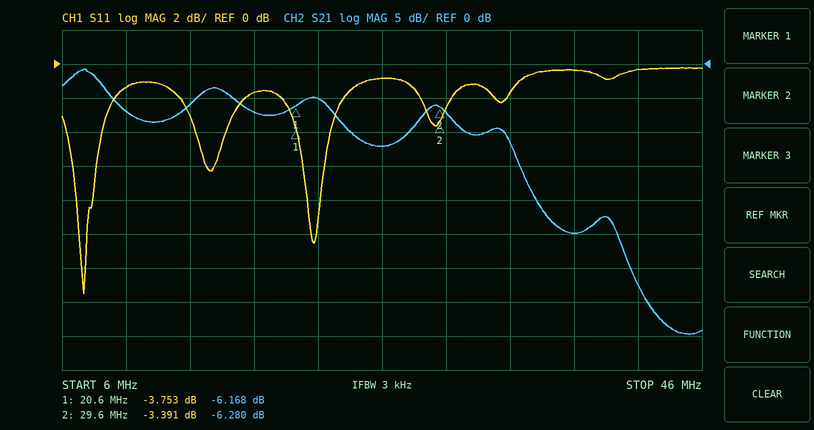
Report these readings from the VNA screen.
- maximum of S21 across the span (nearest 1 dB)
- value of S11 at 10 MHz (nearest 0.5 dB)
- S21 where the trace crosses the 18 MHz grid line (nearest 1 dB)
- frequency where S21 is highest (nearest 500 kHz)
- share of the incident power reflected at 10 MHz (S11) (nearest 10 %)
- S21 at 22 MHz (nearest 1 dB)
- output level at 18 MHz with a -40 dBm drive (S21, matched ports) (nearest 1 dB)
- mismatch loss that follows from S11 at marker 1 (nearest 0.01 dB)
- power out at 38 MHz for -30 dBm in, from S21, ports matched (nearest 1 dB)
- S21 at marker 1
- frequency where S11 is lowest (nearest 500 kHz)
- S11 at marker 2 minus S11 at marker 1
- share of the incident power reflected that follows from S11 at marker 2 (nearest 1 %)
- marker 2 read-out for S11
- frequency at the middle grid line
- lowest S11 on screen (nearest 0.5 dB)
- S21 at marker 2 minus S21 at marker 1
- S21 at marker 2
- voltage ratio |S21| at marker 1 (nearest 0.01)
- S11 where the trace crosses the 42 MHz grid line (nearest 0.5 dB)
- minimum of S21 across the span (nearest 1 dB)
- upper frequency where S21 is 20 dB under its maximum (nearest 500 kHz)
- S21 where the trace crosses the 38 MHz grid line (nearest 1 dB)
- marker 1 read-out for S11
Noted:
-1 dB
-1.5 dB
-7 dB
7.5 MHz
70 %
-5 dB
-47 dBm
2.38 dB
-55 dBm
-6.168 dB
7.5 MHz
0.362 dB
46 %
-3.391 dB
26 MHz
-13.5 dB
-0.112 dB
-6.280 dB
0.49
-0.5 dB
-40 dB
36.0 MHz
-25 dB
-3.753 dB
